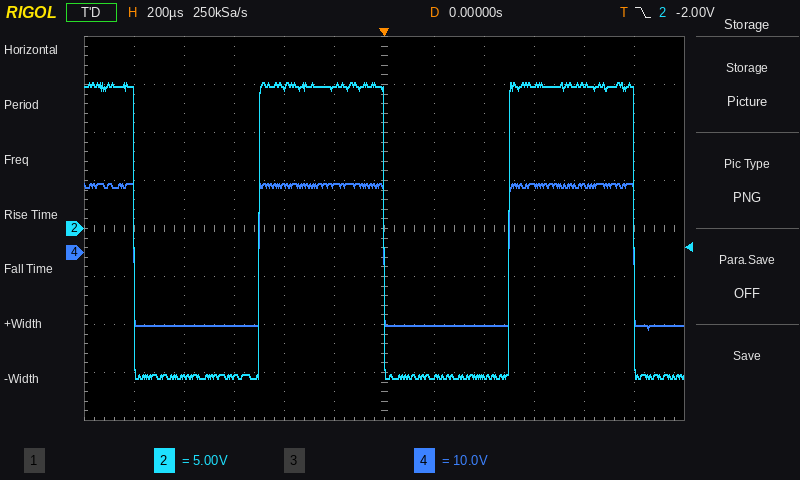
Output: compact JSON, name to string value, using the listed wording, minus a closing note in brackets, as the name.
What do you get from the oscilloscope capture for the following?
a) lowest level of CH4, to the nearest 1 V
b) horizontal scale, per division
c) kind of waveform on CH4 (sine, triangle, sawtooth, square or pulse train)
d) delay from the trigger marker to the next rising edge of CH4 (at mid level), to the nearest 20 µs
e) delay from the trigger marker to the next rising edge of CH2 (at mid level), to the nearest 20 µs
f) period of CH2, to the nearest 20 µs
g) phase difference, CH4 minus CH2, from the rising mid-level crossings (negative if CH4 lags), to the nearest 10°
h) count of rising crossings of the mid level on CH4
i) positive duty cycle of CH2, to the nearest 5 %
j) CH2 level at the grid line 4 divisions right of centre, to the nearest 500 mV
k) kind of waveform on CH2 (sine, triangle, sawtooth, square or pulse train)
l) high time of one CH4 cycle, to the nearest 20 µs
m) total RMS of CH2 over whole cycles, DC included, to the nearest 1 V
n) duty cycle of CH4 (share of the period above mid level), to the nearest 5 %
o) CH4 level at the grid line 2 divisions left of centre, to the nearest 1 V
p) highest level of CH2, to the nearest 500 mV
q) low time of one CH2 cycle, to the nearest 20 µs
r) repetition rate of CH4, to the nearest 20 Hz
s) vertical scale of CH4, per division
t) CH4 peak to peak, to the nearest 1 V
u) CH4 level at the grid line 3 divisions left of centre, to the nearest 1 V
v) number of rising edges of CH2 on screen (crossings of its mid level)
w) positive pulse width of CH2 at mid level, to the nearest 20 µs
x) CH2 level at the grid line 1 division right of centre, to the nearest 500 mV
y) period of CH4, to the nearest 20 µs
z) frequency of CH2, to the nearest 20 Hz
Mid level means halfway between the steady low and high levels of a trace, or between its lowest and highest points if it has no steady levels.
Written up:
{"lowest level of CH4, to the nearest 1 V": "-16 V", "horizontal scale, per division": "200 µs", "kind of waveform on CH4": "square", "delay from the trigger marker to the next rising edge of CH4 (at mid level), to the nearest 20 µs": "500 µs", "delay from the trigger marker to the next rising edge of CH2 (at mid level), to the nearest 20 µs": "500 µs", "period of CH2, to the nearest 20 µs": "1.00 ms", "phase difference, CH4 minus CH2, from the rising mid-level crossings (negative if CH4 lags), to the nearest 10°": "0°", "count of rising crossings of the mid level on CH4": "2", "positive duty cycle of CH2, to the nearest 5 %": "50 %", "CH2 level at the grid line 4 divisions right of centre, to the nearest 500 mV": "15.0 V", "kind of waveform on CH2": "square", "high time of one CH4 cycle, to the nearest 20 µs": "500 µs", "total RMS of CH2 over whole cycles, DC included, to the nearest 1 V": "15 V", "duty cycle of CH4 (share of the period above mid level), to the nearest 5 %": "50 %", "CH4 level at the grid line 2 divisions left of centre, to the nearest 1 V": "14 V", "highest level of CH2, to the nearest 500 mV": "15.0 V", "low time of one CH2 cycle, to the nearest 20 µs": "500 µs", "repetition rate of CH4, to the nearest 20 Hz": "1.00 kHz", "vertical scale of CH4, per division": "10 V", "CH4 peak to peak, to the nearest 1 V": "30 V", "CH4 level at the grid line 3 divisions left of centre, to the nearest 1 V": "-15 V", "number of rising edges of CH2 on screen": "2", "positive pulse width of CH2 at mid level, to the nearest 20 µs": "500 µs", "CH2 level at the grid line 1 division right of centre, to the nearest 500 mV": "-15.5 V", "period of CH4, to the nearest 20 µs": "1.00 ms", "frequency of CH2, to the nearest 20 Hz": "1.00 kHz"}
